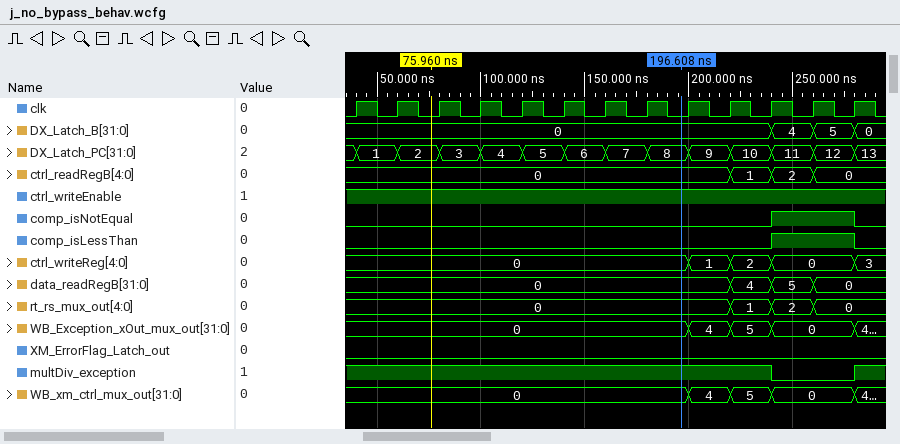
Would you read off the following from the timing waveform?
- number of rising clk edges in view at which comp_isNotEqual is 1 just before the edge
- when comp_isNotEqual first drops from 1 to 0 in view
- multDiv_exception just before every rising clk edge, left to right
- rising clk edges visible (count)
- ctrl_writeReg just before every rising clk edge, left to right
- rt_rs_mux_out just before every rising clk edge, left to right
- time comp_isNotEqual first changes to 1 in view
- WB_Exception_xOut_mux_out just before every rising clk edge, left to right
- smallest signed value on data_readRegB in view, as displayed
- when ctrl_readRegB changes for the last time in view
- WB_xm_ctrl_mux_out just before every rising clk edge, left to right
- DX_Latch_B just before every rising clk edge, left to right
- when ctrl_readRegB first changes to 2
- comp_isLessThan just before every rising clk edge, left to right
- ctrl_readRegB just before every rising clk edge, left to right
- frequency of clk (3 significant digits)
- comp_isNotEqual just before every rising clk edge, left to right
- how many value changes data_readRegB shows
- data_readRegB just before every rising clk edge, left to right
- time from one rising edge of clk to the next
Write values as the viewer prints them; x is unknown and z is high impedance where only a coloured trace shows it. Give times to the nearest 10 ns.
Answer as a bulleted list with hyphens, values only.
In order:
- 2
- 280 ns
- 1 1 1 1 1 1 1 1 1 1 1 0 0
- 13
- 0, 0, 0, 0, 0, 0, 0, 0, 0, 1, 2, 0, 0
- 0, 0, 0, 0, 0, 0, 0, 0, 0, 0, 1, 2, 0
- 240 ns
- 0, 0, 0, 0, 0, 0, 0, 0, 0, 4, 5, 0, 0
- 0
- 260 ns
- 0, 0, 0, 0, 0, 0, 0, 0, 0, 4, 5, 0, 0
- 0, 0, 0, 0, 0, 0, 0, 0, 0, 0, 0, 4, 5
- 240 ns
- 0 0 0 0 0 0 0 0 0 0 0 1 1
- 0, 0, 0, 0, 0, 0, 0, 0, 0, 0, 1, 2, 0
- 50.0 MHz
- 0 0 0 0 0 0 0 0 0 0 0 1 1
- 3
- 0, 0, 0, 0, 0, 0, 0, 0, 0, 0, 4, 5, 0
- 20 ns
